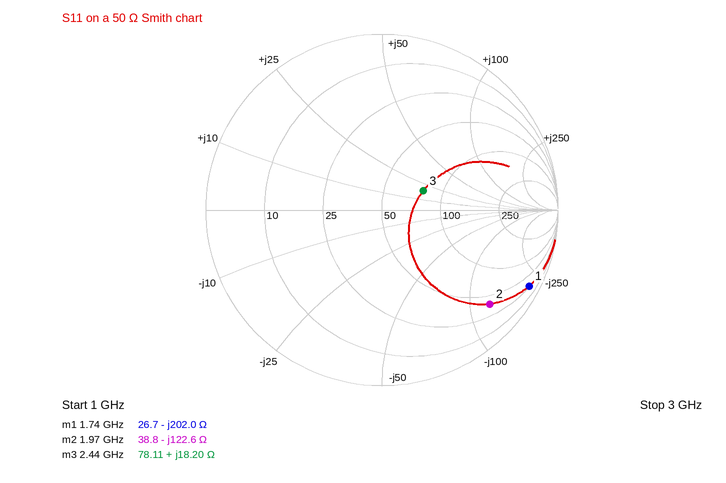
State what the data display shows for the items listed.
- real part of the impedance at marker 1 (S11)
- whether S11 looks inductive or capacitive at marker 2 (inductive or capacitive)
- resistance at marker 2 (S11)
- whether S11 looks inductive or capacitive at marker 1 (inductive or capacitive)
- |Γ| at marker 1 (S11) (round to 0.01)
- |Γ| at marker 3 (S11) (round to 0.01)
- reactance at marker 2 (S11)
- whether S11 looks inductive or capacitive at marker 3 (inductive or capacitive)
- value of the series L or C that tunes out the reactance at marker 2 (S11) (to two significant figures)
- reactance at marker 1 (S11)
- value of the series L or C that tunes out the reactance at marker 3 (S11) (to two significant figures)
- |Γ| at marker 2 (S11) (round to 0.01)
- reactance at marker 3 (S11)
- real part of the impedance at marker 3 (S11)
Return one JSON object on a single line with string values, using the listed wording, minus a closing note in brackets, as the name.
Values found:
{"real part of the impedance at marker 1": "26.7 Ω", "whether S11 looks inductive or capacitive at marker 2": "capacitive", "resistance at marker 2": "38.8 Ω", "whether S11 looks inductive or capacitive at marker 1": "capacitive", "|Γ| at marker 1 (S11)": "0.94", "|Γ| at marker 3 (S11)": "0.26", "reactance at marker 2": "-122.6 Ω", "whether S11 looks inductive or capacitive at marker 3": "inductive", "value of the series L or C that tunes out the reactance at marker 2 (S11)": "9.9 nH", "reactance at marker 1": "-202.0 Ω", "value of the series L or C that tunes out the reactance at marker 3 (S11)": "3.6 pF", "|Γ| at marker 2 (S11)": "0.81", "reactance at marker 3": "+18.20 Ω", "real part of the impedance at marker 3": "78.11 Ω"}
